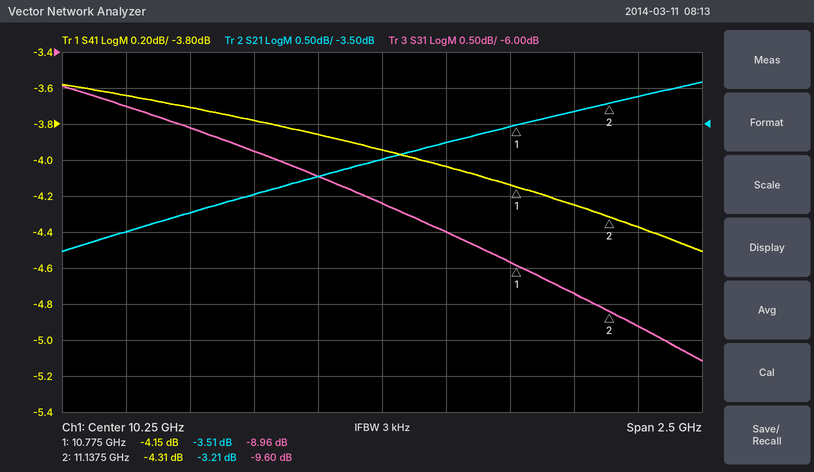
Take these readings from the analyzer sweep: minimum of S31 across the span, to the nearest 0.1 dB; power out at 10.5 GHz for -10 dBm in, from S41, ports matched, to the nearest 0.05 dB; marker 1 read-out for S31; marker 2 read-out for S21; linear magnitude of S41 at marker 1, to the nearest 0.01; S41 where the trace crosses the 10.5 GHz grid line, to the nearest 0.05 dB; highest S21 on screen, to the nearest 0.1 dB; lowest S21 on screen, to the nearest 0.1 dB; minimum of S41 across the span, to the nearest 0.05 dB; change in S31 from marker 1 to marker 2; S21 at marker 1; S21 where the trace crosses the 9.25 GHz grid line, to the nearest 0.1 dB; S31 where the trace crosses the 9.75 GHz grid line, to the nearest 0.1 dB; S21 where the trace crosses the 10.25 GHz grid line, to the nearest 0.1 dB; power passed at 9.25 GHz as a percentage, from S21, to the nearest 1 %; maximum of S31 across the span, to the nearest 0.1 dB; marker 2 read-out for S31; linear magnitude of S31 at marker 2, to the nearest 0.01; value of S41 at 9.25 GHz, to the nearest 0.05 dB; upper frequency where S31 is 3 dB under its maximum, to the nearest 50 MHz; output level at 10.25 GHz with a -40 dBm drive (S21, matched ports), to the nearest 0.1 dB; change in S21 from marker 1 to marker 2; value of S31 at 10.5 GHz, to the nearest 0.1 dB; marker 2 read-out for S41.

-10.3 dB
-14.05 dBm
-8.96 dB
-3.21 dB
0.62
-4.05 dB
-2.9 dB
-5.3 dB
-4.50 dB
-0.64 dB
-3.51 dB
-5.0 dB
-7.4 dB
-4.0 dB
32 %
-6.5 dB
-9.60 dB
0.33
-3.65 dB
11.05 GHz
-44.0 dBm
0.30 dB
-8.5 dB
-4.31 dB
